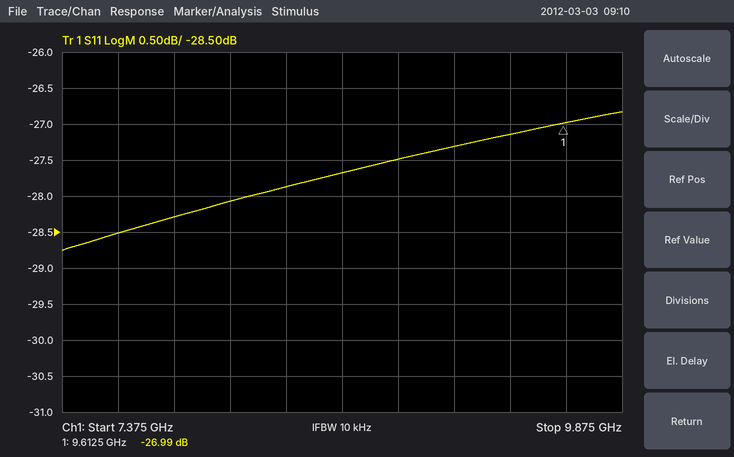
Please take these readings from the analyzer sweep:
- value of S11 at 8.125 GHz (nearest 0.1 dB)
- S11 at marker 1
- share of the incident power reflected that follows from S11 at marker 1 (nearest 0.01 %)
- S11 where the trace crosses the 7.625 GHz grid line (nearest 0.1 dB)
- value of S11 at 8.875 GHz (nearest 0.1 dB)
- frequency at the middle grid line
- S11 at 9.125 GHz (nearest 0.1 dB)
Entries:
-28.1 dB
-26.99 dB
0.20 %
-28.5 dB
-27.5 dB
8.625 GHz
-27.3 dB
